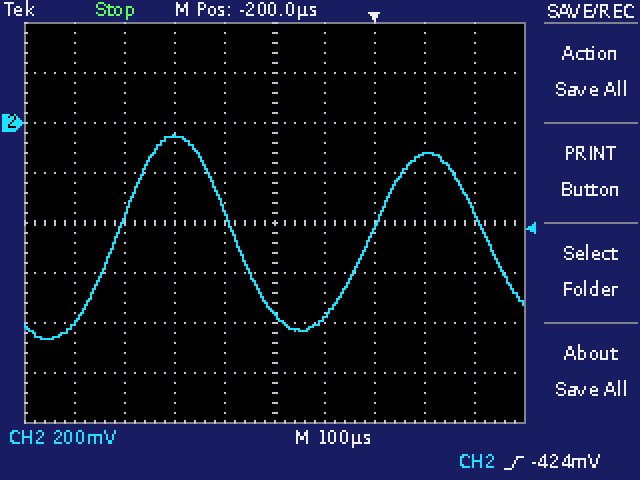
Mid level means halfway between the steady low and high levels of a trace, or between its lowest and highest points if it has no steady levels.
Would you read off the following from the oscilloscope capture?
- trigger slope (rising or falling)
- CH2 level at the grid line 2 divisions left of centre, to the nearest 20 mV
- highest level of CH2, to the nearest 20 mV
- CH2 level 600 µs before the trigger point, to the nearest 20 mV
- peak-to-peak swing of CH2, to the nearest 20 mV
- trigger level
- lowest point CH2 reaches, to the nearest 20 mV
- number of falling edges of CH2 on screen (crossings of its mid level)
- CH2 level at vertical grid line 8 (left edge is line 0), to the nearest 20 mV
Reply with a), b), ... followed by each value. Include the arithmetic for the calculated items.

a) rising
b) -60 mV
c) -40 mV
d) -800 mV
e) -40 mV − (-860 mV) = 820 mV
f) -424 mV
g) -860 mV
h) 2
i) -120 mV
